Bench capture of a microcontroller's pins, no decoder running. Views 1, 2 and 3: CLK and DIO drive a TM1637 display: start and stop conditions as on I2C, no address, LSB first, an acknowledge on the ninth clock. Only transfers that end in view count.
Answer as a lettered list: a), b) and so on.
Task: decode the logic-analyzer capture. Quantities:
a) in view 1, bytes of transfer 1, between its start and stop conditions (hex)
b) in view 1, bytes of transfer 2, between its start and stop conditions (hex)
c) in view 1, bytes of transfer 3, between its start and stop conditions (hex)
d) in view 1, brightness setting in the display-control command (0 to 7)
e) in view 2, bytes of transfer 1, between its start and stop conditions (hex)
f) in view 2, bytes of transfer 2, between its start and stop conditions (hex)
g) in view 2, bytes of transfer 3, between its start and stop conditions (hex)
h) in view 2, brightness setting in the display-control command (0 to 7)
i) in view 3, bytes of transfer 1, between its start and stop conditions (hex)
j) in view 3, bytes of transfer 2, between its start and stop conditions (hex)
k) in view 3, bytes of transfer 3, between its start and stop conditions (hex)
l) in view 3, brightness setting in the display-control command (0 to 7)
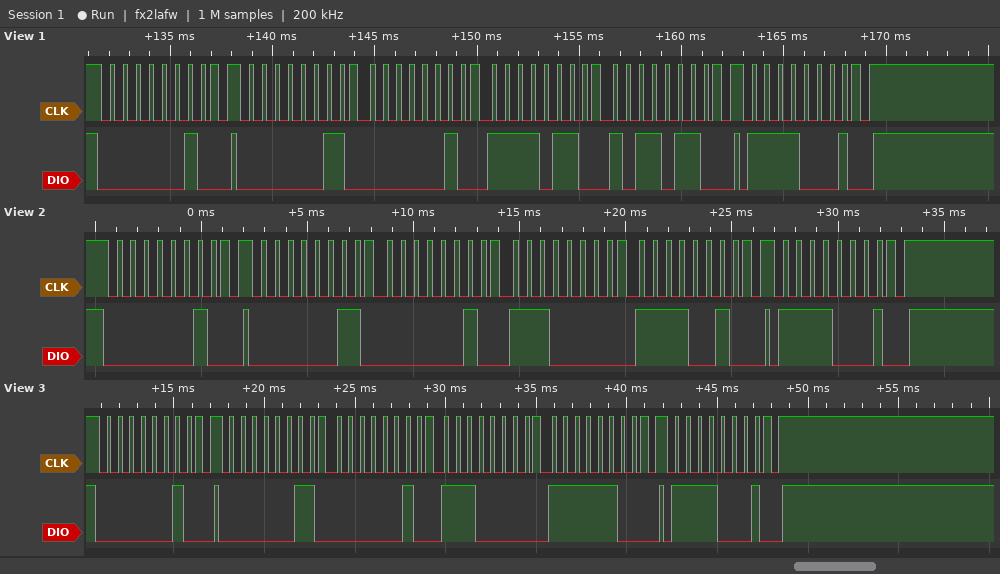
a) 40
b) C0 40 6F 6D
c) 8F
d) 7
e) 40
f) C0 40 07 4F
g) 8F
h) 7
i) 40
j) C0 40 07 3F
k) 8F
l) 7
